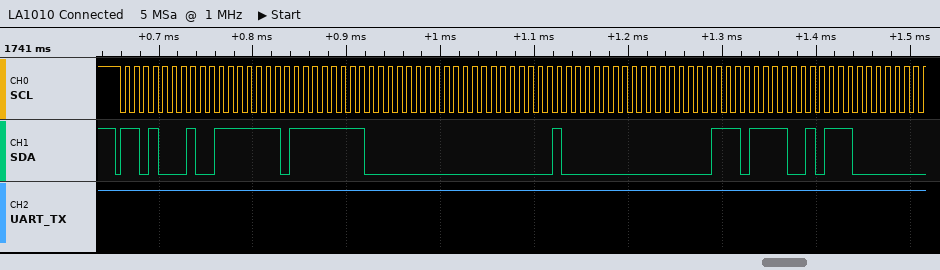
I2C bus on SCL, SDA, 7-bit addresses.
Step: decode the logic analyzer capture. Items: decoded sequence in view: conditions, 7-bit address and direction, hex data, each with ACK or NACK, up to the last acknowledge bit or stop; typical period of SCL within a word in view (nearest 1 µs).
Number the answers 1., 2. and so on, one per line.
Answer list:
1. start, address 68 read ACK, 7F ACK, FF ACK, 00 ACK, 00 ACK, 40 ACK, 00 ACK, EF ACK, 5C ACK
2. 10 µs
